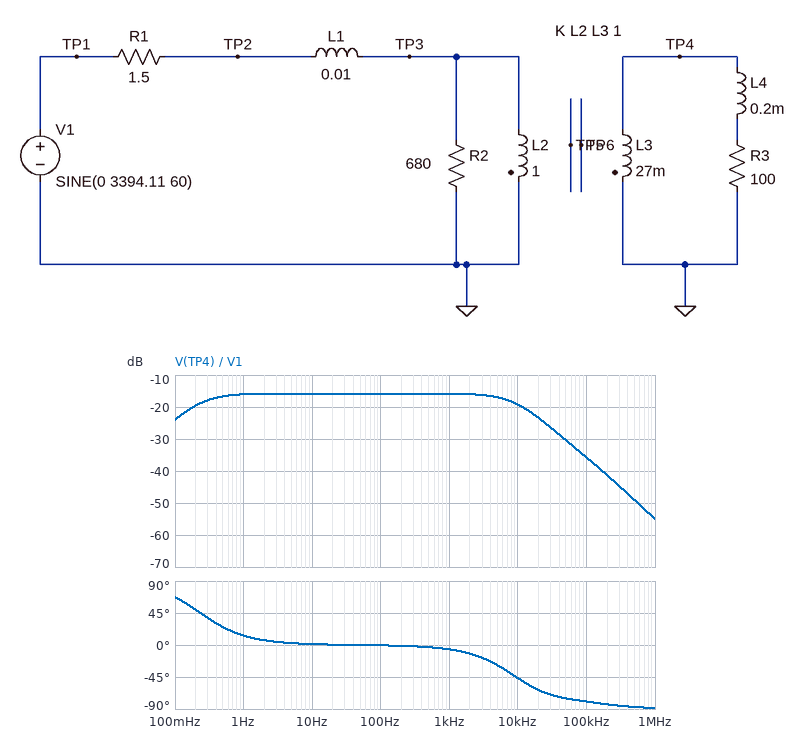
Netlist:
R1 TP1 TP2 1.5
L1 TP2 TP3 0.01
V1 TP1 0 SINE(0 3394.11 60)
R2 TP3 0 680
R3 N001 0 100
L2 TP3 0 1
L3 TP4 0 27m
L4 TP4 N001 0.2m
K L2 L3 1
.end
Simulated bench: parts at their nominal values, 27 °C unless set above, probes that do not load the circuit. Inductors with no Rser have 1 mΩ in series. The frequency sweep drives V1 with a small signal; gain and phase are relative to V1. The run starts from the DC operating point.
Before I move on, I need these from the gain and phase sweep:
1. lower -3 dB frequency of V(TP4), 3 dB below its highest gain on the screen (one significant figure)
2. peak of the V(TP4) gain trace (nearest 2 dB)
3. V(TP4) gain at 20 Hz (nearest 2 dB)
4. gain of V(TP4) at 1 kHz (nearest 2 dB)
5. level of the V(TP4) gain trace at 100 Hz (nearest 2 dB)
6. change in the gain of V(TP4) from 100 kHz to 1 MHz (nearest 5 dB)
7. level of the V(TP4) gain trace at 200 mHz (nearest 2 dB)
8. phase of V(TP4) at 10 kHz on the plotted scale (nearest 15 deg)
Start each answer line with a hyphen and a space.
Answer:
- 200 mHz
- -16 dB
- -16 dB
- -16 dB
- -16 dB
- -20 dB
- -20 dB
- -45 deg
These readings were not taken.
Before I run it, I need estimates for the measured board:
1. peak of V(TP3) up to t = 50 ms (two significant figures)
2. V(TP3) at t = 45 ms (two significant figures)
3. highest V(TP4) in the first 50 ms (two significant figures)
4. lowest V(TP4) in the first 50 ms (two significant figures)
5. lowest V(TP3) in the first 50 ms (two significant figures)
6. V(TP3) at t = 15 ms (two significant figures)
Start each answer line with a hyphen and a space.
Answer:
- 3.3 kV
- -3.2 kV
- 550 V
- -550 V
- -3.4 kV
- -2.0 kV
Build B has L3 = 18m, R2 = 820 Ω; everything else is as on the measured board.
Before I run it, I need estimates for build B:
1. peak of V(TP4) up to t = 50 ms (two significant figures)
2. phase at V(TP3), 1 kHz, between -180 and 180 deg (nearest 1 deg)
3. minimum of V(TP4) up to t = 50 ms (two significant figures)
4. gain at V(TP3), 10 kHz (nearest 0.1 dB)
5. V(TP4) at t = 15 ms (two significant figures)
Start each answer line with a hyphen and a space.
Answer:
- 450 V
- -5 deg
- -450 V
- -2.6 dB
- -270 V
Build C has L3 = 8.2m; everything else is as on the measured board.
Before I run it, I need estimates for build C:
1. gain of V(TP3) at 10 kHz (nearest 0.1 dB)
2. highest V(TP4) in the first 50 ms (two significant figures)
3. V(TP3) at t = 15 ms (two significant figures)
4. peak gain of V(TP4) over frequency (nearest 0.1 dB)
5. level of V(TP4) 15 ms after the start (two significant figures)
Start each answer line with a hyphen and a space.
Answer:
- -3.0 dB
- 300 V
- -2.0 kV
- -21.0 dB
- -180 V
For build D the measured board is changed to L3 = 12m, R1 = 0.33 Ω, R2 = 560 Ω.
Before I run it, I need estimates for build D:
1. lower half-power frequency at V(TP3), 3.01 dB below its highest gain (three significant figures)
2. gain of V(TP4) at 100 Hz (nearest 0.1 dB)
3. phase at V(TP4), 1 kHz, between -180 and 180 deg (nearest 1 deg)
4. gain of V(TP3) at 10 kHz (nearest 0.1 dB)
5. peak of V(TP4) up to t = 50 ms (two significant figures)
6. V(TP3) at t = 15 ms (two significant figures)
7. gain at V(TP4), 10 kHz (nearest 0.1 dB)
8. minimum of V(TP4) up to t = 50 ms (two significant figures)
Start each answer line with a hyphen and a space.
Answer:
- 52.3 mHz
- -19.3 dB
- -7 deg
- -3.9 dB
- 370 V
- -2.0 kV
- -23.1 dB
- -370 V
